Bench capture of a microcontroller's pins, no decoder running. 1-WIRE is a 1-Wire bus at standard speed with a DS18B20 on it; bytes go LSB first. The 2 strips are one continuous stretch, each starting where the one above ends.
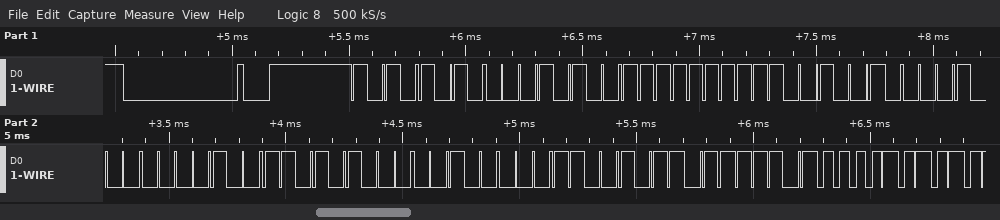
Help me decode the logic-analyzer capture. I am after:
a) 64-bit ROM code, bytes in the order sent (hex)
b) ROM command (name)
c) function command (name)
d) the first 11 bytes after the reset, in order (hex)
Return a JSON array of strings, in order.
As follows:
["28 FF 93 10 90 15 04 D3", "Match ROM", "Read Scratchpad", "55 28 FF 93 10 90 15 04 D3 BE 50"]
